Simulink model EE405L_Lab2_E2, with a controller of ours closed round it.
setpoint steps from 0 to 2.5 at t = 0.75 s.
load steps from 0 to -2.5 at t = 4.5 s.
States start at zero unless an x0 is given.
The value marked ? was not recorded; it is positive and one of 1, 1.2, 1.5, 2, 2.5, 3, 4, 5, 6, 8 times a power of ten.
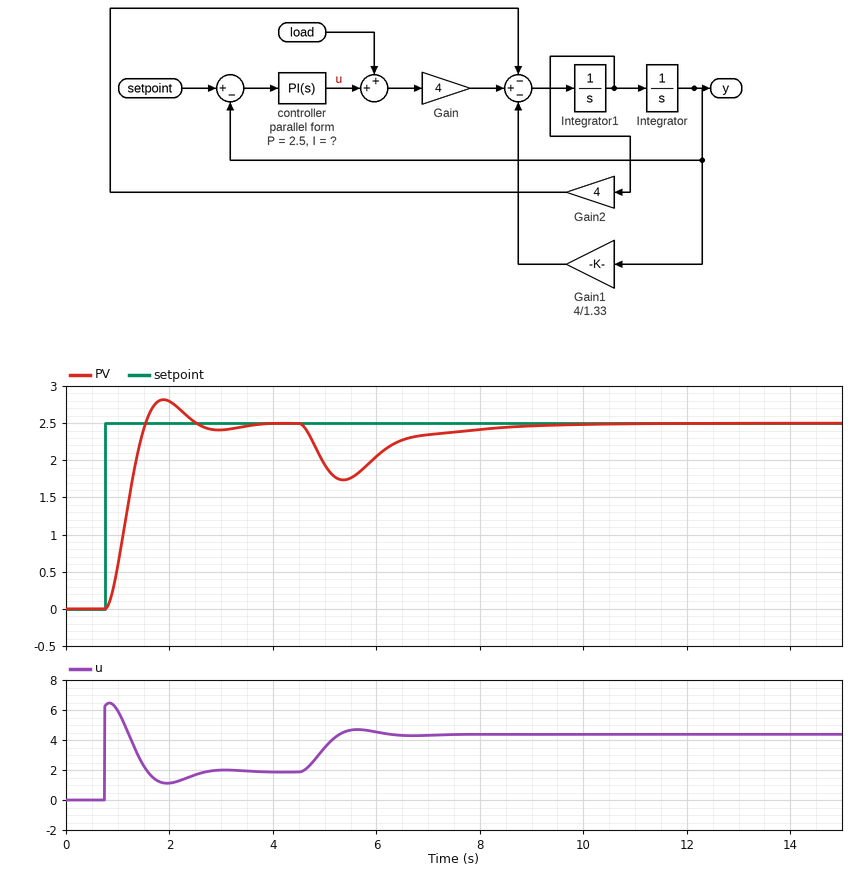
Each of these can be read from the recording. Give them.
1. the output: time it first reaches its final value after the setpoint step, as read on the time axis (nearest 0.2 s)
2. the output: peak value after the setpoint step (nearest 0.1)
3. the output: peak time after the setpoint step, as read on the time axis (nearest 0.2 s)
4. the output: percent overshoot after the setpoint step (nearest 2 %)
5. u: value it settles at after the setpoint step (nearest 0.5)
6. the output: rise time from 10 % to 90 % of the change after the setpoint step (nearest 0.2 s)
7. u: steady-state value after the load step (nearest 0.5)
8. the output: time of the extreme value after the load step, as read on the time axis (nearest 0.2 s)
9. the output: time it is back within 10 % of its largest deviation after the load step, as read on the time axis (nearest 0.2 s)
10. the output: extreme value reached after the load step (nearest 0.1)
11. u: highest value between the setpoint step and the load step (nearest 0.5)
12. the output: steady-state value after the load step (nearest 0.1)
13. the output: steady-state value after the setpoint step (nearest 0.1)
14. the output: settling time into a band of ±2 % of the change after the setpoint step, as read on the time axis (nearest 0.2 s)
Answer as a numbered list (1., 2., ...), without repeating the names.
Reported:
1. 1.6 s
2. 2.8
3. 1.8 s
4. 12 %
5. 2.0
6. 0.6 s
7. 4.5
8. 5.4 s
9. 8.2 s
10. 1.7
11. 6.5
12. 2.5
13. 2.5
14. 3.4 s
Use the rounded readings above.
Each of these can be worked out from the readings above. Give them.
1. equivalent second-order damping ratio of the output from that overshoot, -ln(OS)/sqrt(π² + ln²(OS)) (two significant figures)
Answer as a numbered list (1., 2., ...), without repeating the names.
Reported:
1. 0.56
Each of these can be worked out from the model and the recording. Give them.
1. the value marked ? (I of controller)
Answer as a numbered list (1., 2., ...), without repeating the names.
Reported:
1. 2
